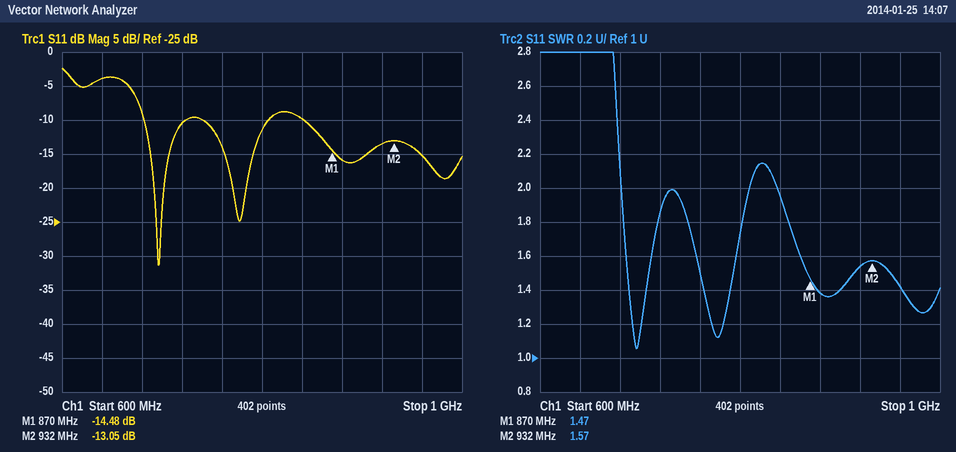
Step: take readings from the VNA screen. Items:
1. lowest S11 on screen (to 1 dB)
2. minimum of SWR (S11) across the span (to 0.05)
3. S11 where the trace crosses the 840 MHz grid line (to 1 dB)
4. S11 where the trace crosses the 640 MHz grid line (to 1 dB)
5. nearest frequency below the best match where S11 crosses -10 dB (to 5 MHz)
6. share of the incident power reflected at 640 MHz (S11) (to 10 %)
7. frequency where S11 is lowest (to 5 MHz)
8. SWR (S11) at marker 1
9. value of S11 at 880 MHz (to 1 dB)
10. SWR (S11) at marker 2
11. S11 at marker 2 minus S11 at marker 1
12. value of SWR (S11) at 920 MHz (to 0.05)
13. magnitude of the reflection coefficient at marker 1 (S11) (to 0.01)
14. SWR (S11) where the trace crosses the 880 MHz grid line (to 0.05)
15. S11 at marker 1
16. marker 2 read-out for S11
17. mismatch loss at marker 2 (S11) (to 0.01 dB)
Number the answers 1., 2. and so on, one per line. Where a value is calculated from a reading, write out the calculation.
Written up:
1. -31 dB
2. 1.05
3. -10 dB
4. -4 dB
5. 680 MHz
6. 10^(-4/10) ≈ 40 %
7. 695 MHz
8. 1.47
9. -16 dB
10. 1.57
11. -13.05 − (-14.48) = 1.43 dB
12. 1.55
13. 10^(-14.48/20) ≈ 0.19
14. 1.40
15. -14.48 dB
16. -13.05 dB
17. −10 log10(1 − 10^(-13.05/10)) ≈ 0.22 dB
